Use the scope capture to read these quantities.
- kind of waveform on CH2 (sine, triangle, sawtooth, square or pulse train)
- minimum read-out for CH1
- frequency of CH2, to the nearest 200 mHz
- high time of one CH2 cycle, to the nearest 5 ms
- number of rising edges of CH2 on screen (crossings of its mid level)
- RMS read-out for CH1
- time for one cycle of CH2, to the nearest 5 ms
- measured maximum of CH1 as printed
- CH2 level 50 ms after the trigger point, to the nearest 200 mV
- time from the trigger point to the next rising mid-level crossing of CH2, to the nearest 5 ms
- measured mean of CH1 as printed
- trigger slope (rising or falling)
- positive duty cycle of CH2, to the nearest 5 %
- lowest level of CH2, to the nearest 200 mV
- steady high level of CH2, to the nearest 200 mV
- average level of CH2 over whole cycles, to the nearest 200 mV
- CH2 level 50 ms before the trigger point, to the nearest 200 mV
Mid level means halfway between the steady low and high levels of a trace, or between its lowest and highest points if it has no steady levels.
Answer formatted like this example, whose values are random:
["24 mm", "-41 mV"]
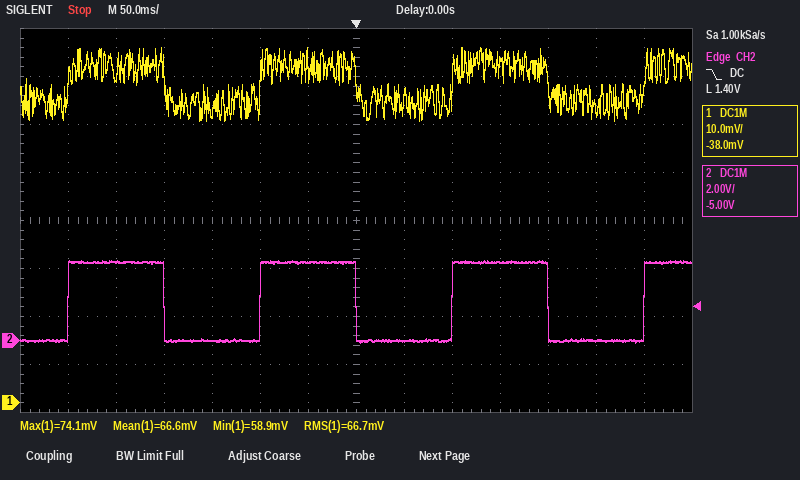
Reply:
["square", "58.9 mV", "5.0 Hz", "100 ms", "4", "66.7 mV", "200 ms", "74.1 mV", "0.0 V", "100 ms", "66.6 mV", "falling", "50 %", "0.0 V", "3.2 V", "1.6 V", "3.2 V"]
